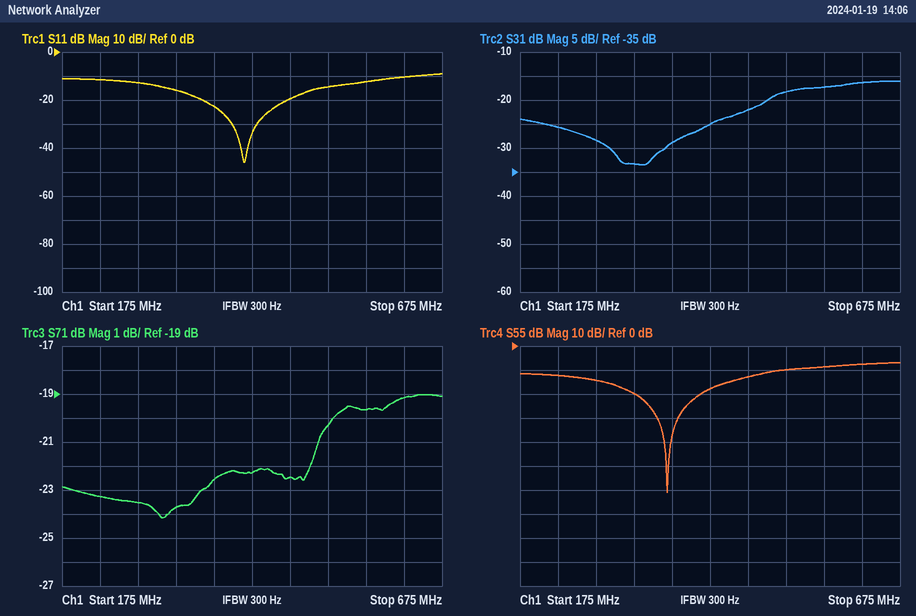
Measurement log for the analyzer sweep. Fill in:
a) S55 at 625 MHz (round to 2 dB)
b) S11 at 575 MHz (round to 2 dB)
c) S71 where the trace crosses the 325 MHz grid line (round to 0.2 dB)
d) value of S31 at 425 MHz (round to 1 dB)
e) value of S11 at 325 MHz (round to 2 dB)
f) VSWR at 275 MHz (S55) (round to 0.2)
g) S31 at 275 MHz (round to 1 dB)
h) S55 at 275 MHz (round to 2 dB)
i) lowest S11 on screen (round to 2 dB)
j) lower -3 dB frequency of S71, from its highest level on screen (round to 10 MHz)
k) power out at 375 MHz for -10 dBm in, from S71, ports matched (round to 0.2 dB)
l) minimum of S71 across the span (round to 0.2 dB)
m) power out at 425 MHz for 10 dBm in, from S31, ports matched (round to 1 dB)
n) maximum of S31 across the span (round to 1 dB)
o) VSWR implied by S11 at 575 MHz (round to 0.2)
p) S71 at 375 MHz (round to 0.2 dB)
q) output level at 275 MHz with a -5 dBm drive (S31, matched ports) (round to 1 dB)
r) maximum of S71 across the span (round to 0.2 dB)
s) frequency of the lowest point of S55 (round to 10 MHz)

-8 dB
-12 dB
-23.8 dB
-25 dB
-16 dB
1.4
-28 dB
-14 dB
-46 dB
500 MHz
-32.6 dBm
-24.2 dB
-15 dBm
-16 dB
1.6
-22.6 dB
-33 dBm
-19.0 dB
370 MHz
